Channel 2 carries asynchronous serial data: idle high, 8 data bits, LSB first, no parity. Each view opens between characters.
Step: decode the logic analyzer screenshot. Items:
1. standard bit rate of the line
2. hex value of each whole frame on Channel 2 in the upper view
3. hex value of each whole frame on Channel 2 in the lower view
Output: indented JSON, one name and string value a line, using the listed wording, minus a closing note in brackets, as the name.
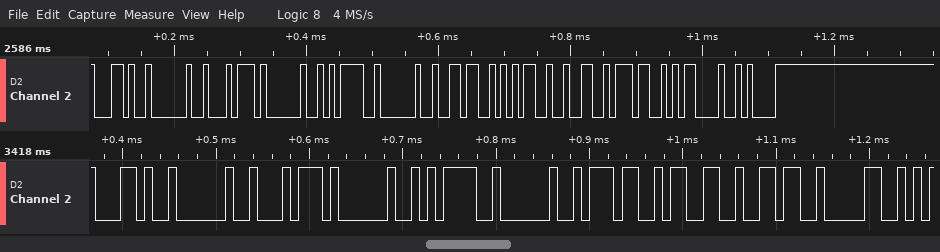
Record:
{
  "standard bit rate of the line": "115200 baud",
  "hex value of each whole frame on Channel 2 in the upper view": "2C, 20, 74, 20, 3D, 20, 36, 35, 32, 37, 0D, 0A",
  "hex value of each whole frame on Channel 2 in the lower view": "2C, 20, 74, 20, 3D, 20, 37, 33, 36, 30"
}
